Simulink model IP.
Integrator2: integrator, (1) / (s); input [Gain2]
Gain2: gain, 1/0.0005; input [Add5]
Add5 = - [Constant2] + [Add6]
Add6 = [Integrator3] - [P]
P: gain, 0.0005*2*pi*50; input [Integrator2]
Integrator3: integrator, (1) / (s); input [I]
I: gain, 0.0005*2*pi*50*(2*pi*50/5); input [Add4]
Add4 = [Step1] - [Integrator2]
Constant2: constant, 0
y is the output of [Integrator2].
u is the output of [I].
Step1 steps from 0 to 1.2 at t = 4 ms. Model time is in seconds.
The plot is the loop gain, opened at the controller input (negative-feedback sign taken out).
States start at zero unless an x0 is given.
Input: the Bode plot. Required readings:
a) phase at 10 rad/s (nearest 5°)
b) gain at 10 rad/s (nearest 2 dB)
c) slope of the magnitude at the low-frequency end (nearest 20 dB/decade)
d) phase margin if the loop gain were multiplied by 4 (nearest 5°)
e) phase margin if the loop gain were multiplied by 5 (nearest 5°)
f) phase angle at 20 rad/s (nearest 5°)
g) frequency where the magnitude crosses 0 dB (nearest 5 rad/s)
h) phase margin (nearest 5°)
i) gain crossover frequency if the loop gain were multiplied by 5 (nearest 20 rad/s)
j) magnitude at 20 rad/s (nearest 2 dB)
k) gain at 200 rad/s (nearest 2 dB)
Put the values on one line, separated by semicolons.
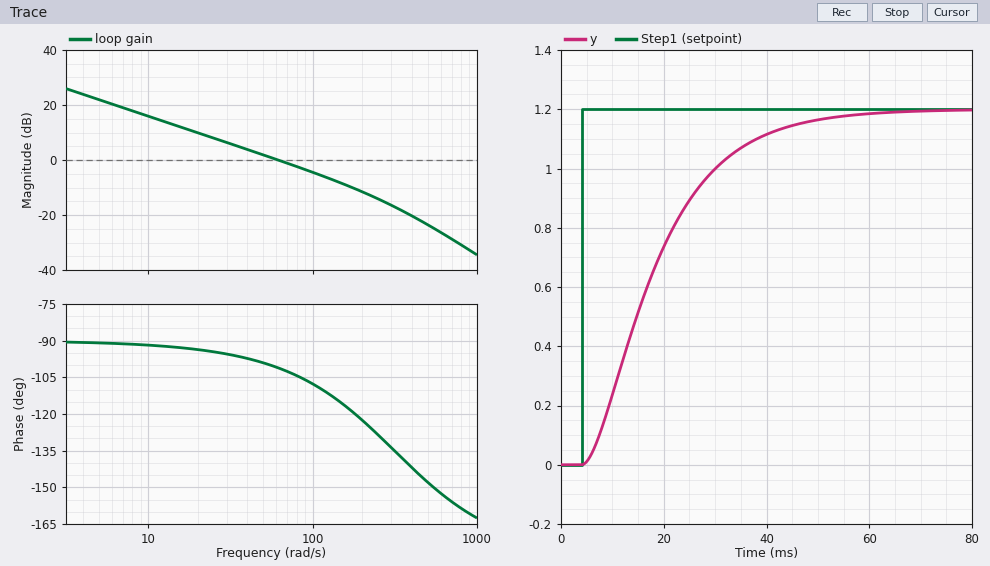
-90°; 16 dB; -20 dB/decade; 55°; 50°; -95°; 60 rad/s; 80°; 240 rad/s; 10 dB; -12 dB
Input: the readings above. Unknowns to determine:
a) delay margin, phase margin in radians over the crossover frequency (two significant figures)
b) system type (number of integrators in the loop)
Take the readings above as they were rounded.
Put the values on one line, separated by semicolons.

0.023 s; 1
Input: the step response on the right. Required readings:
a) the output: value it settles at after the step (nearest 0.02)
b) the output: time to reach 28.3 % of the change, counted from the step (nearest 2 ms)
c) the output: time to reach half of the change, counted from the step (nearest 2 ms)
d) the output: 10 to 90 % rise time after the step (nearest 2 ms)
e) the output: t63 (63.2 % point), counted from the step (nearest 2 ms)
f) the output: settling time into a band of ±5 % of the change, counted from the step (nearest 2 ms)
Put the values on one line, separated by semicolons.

1.20; 8 ms; 12 ms; 28 ms; 16 ms; 40 ms
